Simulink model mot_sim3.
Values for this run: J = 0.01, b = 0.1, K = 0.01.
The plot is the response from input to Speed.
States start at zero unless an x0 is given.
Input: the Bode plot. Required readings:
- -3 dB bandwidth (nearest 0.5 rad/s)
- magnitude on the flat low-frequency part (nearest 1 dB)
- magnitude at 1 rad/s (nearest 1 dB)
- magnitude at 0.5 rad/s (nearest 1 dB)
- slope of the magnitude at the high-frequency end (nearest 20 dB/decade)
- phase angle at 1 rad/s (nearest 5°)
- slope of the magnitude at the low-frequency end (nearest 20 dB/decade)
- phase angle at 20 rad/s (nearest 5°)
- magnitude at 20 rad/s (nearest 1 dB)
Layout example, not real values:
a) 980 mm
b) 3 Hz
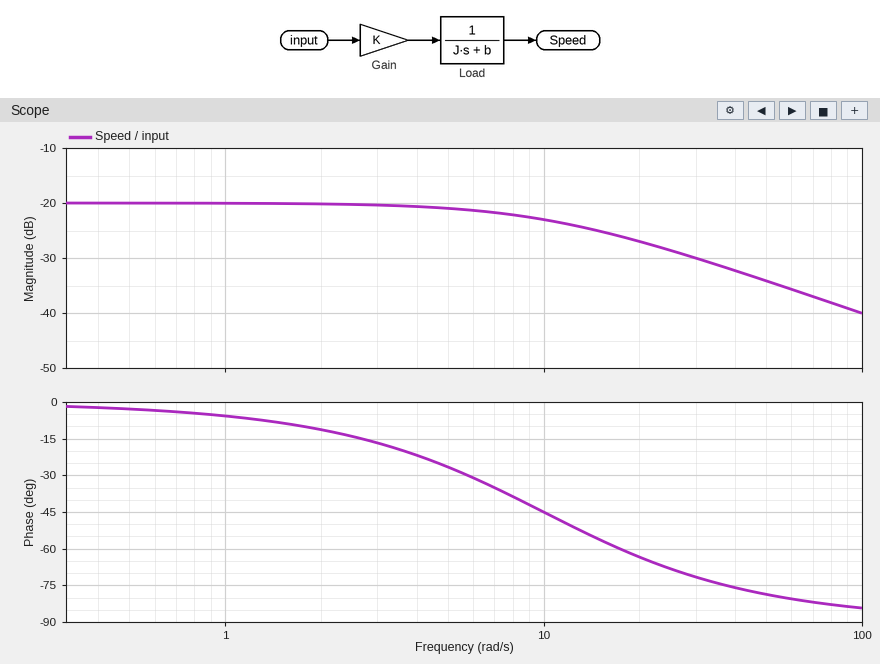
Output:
a) 10.0 rad/s
b) -20 dB
c) -20 dB
d) -20 dB
e) -20 dB/decade
f) -5°
g) 0 dB/decade
h) -65°
i) -27 dB
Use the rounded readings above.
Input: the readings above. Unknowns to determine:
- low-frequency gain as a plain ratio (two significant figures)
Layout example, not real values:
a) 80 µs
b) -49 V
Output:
a) 0.10
